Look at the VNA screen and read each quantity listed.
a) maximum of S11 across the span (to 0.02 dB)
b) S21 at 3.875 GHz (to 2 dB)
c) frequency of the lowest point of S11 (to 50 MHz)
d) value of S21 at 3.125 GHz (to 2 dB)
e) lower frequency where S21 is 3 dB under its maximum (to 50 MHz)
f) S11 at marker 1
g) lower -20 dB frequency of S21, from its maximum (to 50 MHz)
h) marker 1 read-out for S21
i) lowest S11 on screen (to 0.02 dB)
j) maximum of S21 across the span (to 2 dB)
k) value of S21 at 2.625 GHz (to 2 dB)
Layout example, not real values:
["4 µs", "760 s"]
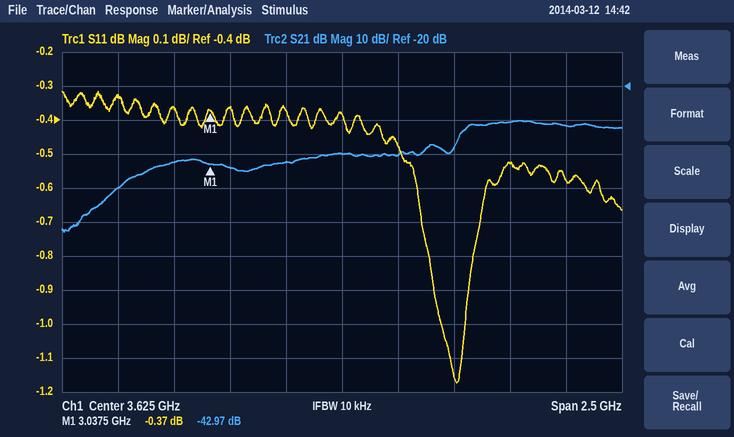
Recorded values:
["-0.32 dB", "-40 dB", "4.15 GHz", "-44 dB", "4.15 GHz", "-0.37 dB", "2.60 GHz", "-42.97 dB", "-1.18 dB", "-30 dB", "-50 dB"]
